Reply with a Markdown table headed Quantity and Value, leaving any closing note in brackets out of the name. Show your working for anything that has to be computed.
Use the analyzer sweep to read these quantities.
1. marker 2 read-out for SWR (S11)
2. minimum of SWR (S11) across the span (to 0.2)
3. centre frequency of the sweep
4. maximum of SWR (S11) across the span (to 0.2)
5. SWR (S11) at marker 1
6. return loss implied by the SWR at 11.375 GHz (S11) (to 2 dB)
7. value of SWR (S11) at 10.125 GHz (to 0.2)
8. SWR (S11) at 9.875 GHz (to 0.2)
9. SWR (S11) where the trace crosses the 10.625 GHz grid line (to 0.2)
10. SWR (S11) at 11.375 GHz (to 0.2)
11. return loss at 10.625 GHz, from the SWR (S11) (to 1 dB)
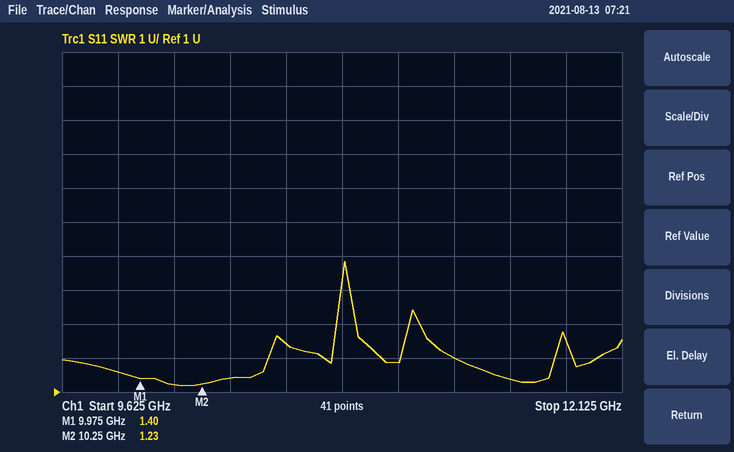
| Quantity | Value |
|---|---|
| marker 2 read-out for SWR | 1.23 |
| minimum of SWR (S11) across the span | 1.2 |
| centre frequency of the sweep | 10.875 GHz |
| maximum of SWR (S11) across the span | 4.8 |
| SWR (S11) at marker 1 | 1.40 |
| return loss implied by the SWR at 11.375 GHz (S11) | −20 log10((2 − 1)/(2 + 1)) ≈ 10 dB |
| value of SWR (S11) at 10.125 GHz | 1.2 |
| SWR (S11) at 9.875 GHz | 1.6 |
| SWR (S11) where the trace crosses the 10.625 GHz grid line | 2.4 |
| SWR (S11) at 11.375 GHz | 2.0 |
| return loss at 10.625 GHz, from the SWR (S11) | −20 log10((2.4 − 1)/(2.4 + 1)) ≈ 8 dB |
